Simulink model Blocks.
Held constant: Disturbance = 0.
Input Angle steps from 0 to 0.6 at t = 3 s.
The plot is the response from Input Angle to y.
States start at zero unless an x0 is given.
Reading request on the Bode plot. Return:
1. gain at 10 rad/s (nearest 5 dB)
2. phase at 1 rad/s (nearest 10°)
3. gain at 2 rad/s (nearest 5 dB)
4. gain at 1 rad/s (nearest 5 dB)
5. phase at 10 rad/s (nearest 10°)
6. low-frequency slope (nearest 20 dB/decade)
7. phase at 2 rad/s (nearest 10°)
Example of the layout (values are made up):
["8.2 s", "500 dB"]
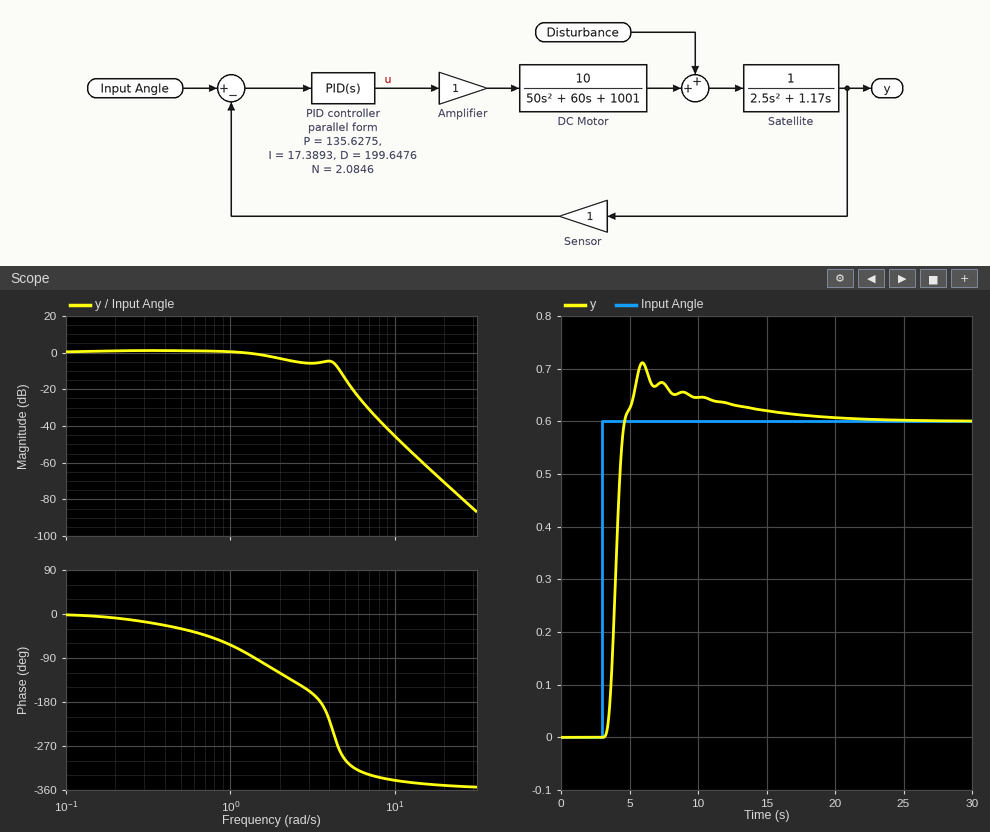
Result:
["-45 dB", "-60°", "-5 dB", "0 dB", "-340°", "0 dB/decade", "-120°"]
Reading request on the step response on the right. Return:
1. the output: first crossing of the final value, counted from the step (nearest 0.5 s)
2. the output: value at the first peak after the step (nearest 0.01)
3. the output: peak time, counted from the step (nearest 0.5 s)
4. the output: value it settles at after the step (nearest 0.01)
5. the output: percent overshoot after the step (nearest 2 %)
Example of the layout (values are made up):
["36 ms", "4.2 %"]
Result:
["1.5 s", "0.71", "3.0 s", "0.60", "18 %"]
